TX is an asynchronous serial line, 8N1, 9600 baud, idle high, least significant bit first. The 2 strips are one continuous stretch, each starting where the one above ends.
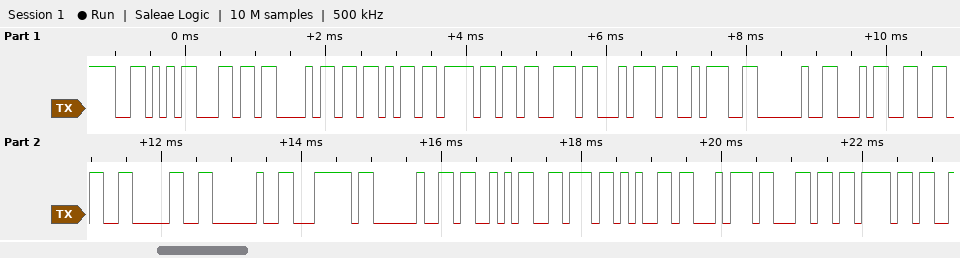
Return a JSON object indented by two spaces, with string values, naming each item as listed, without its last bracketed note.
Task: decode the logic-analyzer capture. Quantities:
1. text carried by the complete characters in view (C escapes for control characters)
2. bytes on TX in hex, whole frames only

{
  "text carried by the complete characters in view": "\"Vlhkost: 460 | Svetlo\"",
  "bytes on TX in hex, whole frames only": "56 6C 68 6B 6F 73 74 3A 20 34 36 30 20 7C 20 53 76 65 74 6C 6F"
}
